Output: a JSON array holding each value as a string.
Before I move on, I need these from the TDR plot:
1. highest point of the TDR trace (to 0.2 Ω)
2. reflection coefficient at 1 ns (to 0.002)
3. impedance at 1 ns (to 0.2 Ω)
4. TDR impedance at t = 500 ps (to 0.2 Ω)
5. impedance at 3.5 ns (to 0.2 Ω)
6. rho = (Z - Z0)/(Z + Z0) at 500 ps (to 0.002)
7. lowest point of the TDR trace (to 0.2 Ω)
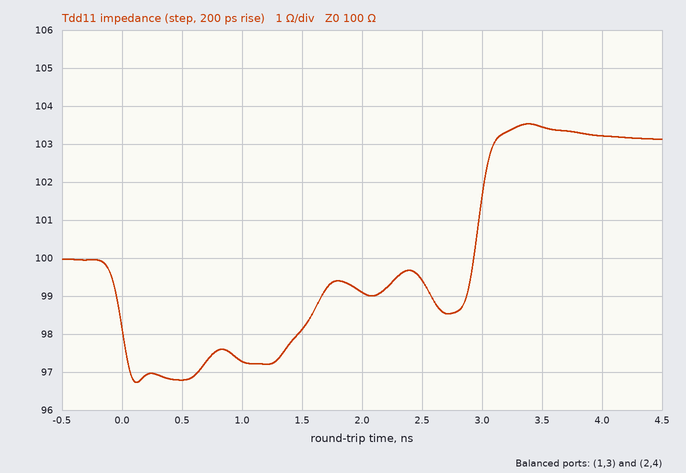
["103.6 Ω", "-0.014", "97.2 Ω", "96.8 Ω", "103.4 Ω", "-0.016", "96.8 Ω"]
